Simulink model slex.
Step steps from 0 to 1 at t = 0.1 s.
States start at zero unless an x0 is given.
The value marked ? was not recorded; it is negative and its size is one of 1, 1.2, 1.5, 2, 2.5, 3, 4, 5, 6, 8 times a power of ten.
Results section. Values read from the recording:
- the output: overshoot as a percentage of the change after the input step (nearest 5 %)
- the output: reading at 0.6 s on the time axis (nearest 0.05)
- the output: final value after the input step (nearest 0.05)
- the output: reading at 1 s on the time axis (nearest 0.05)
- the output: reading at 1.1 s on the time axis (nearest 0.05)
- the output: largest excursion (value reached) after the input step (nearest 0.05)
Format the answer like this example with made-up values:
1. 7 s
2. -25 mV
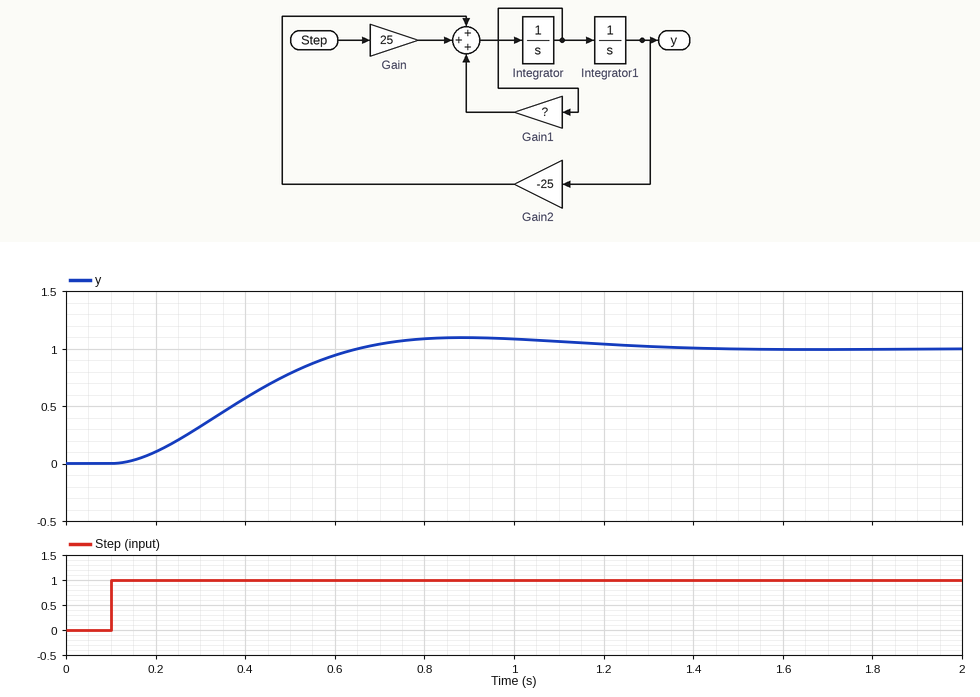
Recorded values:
1. 10 %
2. 0.95
3. 1.00
4. 1.10
5. 1.05
6. 1.10
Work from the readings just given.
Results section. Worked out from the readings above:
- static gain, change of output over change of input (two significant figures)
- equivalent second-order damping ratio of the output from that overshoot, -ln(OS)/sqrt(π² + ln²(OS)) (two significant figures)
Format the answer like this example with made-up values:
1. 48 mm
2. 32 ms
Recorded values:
1. 1.0
2. 0.59
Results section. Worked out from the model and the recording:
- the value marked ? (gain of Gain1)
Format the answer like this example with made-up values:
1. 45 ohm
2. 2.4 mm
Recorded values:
1. -6
